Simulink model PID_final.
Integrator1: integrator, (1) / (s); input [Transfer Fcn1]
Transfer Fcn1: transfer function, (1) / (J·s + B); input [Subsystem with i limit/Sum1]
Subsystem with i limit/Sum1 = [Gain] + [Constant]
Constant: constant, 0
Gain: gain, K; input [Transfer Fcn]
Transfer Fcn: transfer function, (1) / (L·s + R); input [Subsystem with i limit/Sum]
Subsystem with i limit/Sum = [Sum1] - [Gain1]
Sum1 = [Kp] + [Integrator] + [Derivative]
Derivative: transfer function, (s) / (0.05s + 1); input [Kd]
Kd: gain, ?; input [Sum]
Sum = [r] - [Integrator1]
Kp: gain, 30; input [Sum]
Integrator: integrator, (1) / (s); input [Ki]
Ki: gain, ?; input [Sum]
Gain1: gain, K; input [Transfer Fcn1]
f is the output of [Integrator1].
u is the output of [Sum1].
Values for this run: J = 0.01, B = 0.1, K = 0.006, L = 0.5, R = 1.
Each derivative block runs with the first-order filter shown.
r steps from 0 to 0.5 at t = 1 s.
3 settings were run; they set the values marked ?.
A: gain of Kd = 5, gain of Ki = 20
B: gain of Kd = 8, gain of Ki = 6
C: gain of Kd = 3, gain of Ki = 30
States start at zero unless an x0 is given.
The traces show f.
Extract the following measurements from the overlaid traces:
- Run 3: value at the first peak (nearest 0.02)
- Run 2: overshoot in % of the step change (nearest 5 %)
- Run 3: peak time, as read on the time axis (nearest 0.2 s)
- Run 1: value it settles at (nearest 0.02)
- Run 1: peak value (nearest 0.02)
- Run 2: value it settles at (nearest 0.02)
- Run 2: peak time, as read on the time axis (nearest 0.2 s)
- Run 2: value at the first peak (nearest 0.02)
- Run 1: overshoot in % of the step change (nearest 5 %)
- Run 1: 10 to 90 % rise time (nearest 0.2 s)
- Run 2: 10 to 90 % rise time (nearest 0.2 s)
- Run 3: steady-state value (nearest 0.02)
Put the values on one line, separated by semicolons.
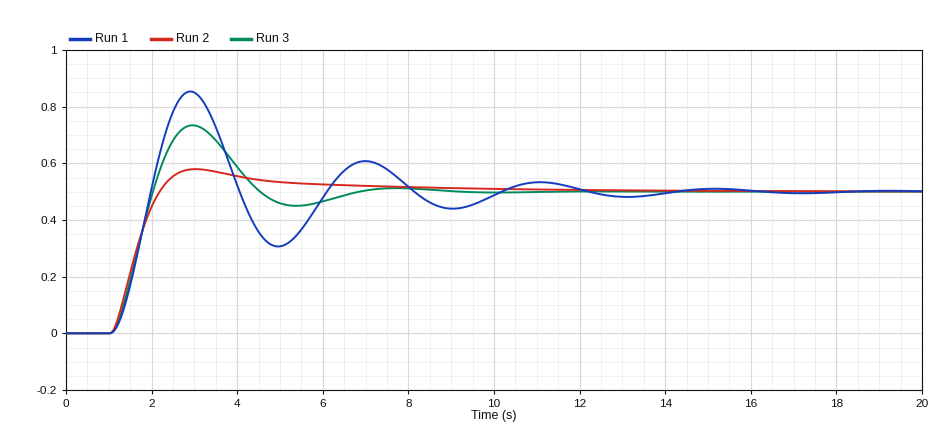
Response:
0.74; 15 %; 3.0 s; 0.50; 0.86; 0.50; 3.0 s; 0.58; 70 %; 0.6 s; 0.8 s; 0.50
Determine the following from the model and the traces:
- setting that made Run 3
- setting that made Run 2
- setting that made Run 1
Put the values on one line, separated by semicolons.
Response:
A; B; C
